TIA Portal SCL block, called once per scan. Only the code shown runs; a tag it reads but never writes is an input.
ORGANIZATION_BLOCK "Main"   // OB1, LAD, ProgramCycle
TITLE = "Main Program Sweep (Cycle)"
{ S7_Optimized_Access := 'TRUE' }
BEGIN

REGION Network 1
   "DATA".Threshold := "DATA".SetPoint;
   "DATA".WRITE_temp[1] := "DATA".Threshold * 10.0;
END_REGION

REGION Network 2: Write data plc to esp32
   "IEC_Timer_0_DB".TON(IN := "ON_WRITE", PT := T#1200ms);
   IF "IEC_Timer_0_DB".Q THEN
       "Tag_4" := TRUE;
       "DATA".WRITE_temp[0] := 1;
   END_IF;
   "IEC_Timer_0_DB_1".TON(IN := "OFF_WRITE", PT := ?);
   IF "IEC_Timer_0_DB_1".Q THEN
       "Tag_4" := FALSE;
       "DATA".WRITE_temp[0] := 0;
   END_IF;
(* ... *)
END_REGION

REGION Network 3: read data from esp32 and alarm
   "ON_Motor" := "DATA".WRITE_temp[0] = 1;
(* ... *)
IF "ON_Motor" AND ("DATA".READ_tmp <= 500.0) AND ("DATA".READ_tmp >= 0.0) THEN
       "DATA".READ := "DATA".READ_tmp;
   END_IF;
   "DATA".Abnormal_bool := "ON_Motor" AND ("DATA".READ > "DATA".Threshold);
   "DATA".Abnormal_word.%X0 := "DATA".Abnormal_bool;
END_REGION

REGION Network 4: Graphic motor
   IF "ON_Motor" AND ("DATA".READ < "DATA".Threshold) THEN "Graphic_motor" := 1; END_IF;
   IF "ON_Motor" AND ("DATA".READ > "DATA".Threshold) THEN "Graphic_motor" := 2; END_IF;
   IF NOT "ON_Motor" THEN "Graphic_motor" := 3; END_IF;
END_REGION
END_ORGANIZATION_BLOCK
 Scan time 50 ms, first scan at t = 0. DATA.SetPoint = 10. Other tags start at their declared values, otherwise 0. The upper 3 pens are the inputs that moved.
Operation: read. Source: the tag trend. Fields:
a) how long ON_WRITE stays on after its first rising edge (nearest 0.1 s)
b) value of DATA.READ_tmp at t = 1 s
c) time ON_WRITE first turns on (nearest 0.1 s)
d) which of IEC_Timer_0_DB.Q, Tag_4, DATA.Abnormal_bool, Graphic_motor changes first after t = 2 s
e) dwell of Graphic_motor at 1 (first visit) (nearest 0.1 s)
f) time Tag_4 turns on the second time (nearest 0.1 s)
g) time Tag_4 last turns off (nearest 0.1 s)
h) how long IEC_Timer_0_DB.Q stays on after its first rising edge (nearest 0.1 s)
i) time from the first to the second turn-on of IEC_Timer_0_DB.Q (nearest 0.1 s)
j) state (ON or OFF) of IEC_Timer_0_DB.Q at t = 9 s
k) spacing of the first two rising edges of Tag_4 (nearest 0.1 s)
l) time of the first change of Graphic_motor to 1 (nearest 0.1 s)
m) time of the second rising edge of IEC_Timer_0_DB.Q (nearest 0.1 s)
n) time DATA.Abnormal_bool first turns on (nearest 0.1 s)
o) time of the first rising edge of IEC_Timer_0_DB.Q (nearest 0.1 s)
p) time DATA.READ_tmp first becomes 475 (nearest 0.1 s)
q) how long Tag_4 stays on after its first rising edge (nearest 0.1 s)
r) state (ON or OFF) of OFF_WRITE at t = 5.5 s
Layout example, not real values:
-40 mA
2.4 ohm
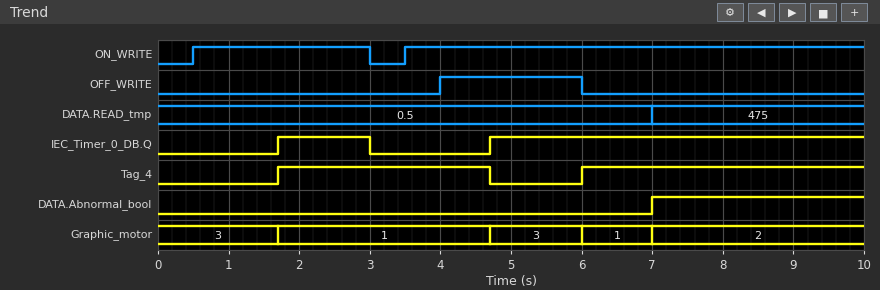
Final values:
2.5 s
0.5
0.5 s
IEC_Timer_0_DB.Q
3.0 s
6.0 s
4.7 s
1.3 s
3.0 s
ON
4.3 s
1.7 s
4.7 s
7.0 s
1.7 s
7.0 s
3.0 s
ON
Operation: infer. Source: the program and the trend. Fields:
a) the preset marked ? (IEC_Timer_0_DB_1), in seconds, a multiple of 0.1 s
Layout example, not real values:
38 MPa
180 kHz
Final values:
0.7 s
